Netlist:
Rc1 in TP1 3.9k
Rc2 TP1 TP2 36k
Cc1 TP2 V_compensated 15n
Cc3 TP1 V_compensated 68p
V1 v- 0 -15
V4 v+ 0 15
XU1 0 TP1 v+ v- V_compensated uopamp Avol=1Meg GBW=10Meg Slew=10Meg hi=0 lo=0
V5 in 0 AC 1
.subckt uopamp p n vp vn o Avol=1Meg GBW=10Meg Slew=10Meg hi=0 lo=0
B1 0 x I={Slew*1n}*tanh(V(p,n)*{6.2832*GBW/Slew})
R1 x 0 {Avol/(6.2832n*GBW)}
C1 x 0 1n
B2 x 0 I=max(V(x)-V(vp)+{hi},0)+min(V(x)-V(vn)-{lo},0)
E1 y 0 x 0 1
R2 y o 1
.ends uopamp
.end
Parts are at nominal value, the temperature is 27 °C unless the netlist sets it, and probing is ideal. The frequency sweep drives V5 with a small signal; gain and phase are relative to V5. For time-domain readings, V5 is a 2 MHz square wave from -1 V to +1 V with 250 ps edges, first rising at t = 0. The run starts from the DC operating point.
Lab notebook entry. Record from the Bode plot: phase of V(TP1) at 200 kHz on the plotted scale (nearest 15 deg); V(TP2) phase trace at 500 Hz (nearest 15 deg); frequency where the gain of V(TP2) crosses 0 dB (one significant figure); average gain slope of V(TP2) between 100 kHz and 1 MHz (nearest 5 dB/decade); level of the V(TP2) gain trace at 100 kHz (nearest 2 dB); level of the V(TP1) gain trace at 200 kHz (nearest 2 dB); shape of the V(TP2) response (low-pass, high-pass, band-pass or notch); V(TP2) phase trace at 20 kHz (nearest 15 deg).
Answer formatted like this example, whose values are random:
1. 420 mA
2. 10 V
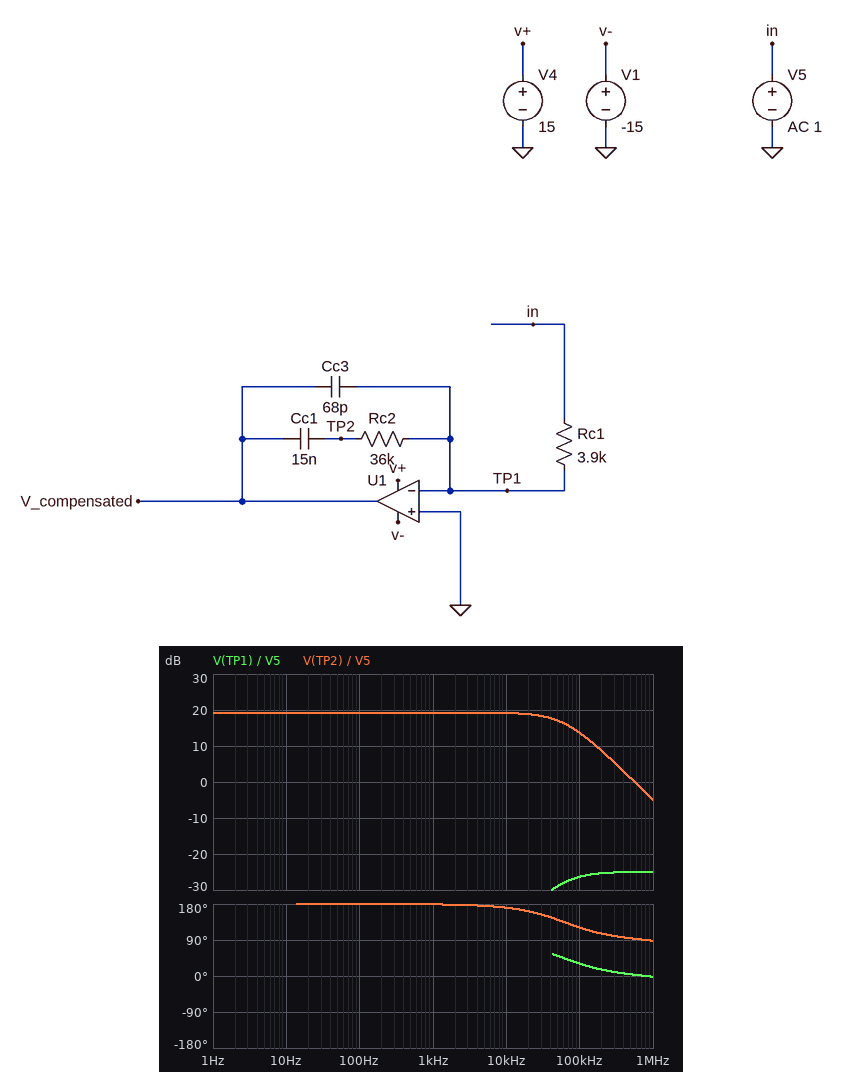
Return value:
1. 15 deg
2. 180 deg
3. 600 kHz
4. -20 dB/decade
5. 14 dB
6. -26 dB
7. low-pass
8. 165 deg
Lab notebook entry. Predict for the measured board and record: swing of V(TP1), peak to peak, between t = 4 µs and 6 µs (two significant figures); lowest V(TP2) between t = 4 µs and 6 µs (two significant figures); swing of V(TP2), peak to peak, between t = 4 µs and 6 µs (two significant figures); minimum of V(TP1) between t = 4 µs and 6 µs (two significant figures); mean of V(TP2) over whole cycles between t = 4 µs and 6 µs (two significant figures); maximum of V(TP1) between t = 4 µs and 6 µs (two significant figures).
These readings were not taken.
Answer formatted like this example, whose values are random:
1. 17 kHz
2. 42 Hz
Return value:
1. 490 mV
2. -1.4 V
3. 420 mV
4. -440 mV
5. -1.1 V
6. 50 mV
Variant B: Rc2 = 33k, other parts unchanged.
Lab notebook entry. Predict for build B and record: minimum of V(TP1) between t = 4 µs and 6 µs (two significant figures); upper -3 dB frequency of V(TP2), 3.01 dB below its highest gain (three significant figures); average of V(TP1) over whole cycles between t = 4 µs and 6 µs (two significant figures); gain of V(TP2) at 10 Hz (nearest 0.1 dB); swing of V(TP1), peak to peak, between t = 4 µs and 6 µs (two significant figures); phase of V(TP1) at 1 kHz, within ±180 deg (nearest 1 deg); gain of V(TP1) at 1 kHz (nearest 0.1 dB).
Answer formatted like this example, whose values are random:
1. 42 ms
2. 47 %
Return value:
1. -450 mV
2. 67.2 kHz
3. -120 mV
4. 18.5 dB
5. 500 mV
6. 71 deg
7. -61.1 dB
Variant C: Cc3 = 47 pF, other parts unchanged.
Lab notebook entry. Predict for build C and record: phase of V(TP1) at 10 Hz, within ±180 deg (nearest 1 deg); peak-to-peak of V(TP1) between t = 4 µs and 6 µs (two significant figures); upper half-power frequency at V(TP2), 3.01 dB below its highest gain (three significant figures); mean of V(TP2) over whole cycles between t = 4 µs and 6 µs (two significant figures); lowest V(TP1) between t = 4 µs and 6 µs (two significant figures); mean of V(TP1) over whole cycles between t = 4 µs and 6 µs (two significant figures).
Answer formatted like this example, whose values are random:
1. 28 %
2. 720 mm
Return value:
1. -43 deg
2. 610 mV
3. 86.8 kHz
4. -1.2 V
5. -530 mV
6. -120 mV
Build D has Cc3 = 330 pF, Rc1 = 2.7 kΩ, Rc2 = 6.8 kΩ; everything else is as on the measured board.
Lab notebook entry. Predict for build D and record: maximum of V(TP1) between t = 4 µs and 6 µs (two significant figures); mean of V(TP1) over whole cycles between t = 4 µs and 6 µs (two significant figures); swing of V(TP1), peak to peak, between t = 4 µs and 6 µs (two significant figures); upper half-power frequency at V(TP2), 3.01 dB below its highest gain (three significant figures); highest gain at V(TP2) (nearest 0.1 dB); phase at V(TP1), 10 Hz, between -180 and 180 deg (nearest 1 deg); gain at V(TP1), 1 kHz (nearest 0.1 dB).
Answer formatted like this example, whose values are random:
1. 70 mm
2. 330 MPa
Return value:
1. -140 mV
2. -280 mV
3. 280 mV
4. 71.2 kHz
5. 7.8 dB
6. -45 deg
7. -66.8 dB
